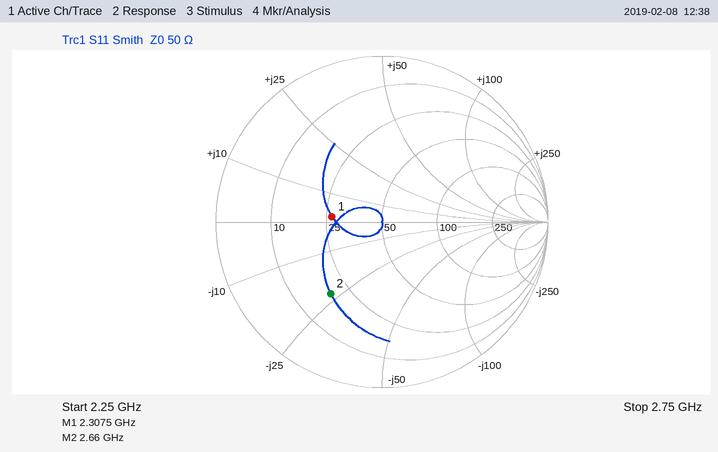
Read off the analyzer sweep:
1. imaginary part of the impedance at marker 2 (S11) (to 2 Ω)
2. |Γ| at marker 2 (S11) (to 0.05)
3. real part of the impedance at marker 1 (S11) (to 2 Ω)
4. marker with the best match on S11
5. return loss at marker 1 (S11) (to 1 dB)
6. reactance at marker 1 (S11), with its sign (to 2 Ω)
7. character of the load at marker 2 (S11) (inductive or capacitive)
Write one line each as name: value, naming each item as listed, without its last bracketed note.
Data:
imaginary part of the impedance at marker 2 (S11): -22 Ω
|Γ| at marker 2 (S11): 0.55
real part of the impedance at marker 1 (S11): 26 Ω
marker with the best match on S11: marker 1
return loss at marker 1 (S11): 10 dB
reactance at marker 1 (S11), with its sign: +2 Ω
character of the load at marker 2 (S11): capacitive
